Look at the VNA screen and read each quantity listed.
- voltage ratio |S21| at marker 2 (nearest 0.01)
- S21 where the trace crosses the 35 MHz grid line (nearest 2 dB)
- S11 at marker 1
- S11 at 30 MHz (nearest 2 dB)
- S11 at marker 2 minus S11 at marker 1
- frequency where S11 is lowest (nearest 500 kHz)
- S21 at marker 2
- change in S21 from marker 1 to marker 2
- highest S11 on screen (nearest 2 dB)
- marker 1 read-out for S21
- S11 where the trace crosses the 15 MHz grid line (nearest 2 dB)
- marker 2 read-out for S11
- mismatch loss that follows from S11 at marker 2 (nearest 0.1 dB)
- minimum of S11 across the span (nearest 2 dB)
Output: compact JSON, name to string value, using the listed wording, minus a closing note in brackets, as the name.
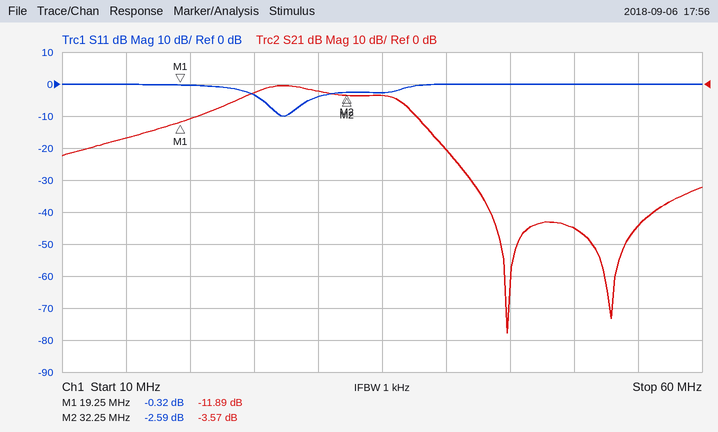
{"voltage ratio |S21| at marker 2": "0.66", "S21 where the trace crosses the 35 MHz grid line": "-4 dB", "S11 at marker 1": "-0.32 dB", "S11 at 30 MHz": "-4 dB", "S11 at marker 2 minus S11 at marker 1": "-2.27 dB", "frequency where S11 is lowest": "27.5 MHz", "S21 at marker 2": "-3.57 dB", "change in S21 from marker 1 to marker 2": "8.32 dB", "highest S11 on screen": "0 dB", "marker 1 read-out for S21": "-11.89 dB", "S11 where the trace crosses the 15 MHz grid line": "0 dB", "marker 2 read-out for S11": "-2.59 dB", "mismatch loss that follows from S11 at marker 2": "3.5 dB", "minimum of S11 across the span": "-10 dB"}
